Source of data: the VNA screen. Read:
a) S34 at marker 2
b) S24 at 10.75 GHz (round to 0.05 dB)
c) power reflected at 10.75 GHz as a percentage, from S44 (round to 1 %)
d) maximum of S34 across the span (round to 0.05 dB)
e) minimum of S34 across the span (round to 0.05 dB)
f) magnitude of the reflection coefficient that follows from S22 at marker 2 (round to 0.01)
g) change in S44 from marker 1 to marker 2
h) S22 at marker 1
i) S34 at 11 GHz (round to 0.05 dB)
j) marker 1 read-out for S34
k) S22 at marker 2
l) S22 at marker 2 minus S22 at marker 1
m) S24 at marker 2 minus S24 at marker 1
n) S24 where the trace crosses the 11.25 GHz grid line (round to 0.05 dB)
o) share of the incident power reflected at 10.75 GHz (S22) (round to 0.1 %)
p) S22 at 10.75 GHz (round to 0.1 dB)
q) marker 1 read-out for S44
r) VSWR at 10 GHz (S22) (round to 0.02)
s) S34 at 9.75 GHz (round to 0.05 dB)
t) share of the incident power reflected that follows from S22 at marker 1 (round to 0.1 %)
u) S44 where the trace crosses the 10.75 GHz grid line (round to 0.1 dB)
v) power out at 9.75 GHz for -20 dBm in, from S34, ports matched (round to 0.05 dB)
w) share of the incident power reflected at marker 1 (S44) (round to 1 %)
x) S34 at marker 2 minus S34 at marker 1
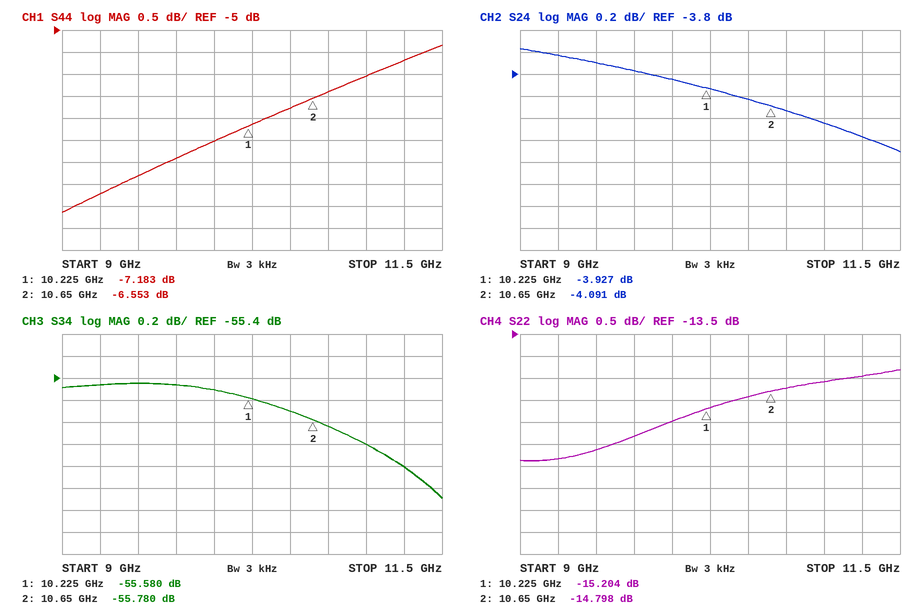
-55.780 dB
-4.15 dB
23 %
-55.45 dB
-56.50 dB
0.18
0.630 dB
-15.204 dB
-56.00 dB
-55.580 dB
-14.798 dB
0.406 dB
-0.164 dB
-4.35 dB
3.4 %
-14.7 dB
-7.183 dB
1.40
-55.45 dB
3.0 %
-6.4 dB
-75.45 dBm
19 %
-0.200 dB
